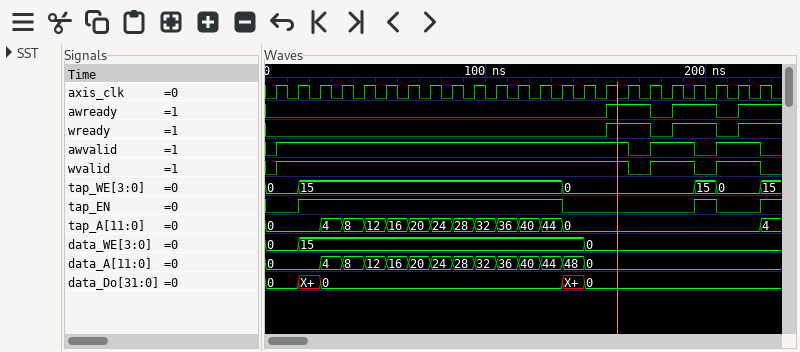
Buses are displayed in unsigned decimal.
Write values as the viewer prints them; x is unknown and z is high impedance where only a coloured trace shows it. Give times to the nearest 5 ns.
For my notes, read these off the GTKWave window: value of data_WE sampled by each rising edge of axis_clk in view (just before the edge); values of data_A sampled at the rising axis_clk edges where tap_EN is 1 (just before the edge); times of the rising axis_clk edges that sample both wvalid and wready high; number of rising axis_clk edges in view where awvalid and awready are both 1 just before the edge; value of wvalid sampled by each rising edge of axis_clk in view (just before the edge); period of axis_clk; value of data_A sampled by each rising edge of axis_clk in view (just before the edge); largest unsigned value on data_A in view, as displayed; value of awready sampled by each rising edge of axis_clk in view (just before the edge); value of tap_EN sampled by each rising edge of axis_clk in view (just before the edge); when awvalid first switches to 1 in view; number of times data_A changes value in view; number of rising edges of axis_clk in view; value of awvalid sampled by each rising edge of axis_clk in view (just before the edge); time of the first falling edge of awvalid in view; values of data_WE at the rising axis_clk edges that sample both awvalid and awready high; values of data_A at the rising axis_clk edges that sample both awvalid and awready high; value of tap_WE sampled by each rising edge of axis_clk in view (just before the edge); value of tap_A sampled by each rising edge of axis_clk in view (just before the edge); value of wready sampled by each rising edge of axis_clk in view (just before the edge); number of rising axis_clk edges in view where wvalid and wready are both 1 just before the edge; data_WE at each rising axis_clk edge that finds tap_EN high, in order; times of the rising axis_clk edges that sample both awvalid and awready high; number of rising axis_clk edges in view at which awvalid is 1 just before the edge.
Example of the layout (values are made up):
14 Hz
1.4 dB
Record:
0, 0, 15, 15, 15, 15, 15, 15, 15, 15, 15, 15, 15, 15, 15, 0, 0, 0, 0, 0, 0, 0, 0
0, 4, 8, 12, 16, 20, 24, 28, 32, 36, 40, 44, 0
165 ns, 195 ns, 225 ns
3
0 1 1 1 1 1 1 1 1 1 1 1 1 1 1 1 1 0 1 1 0 1 1
10 ns
0, 0, 0, 4, 8, 12, 16, 20, 24, 28, 32, 36, 40, 44, 48, 0, 0, 0, 0, 0, 0, 0, 0
48
0 0 0 0 0 0 0 0 0 0 0 0 0 0 0 0 1 1 0 1 1 0 1
0 0 1 1 1 1 1 1 1 1 1 1 1 1 0 0 0 0 0 0 1 0 0
5 ns
13
23
0 1 1 1 1 1 1 1 1 1 1 1 1 1 1 1 1 0 1 1 0 1 1
165 ns
0, 0, 0
0, 0, 0
0, 0, 15, 15, 15, 15, 15, 15, 15, 15, 15, 15, 15, 15, 0, 0, 0, 0, 0, 0, 15, 0, 0
0, 0, 0, 4, 8, 12, 16, 20, 24, 28, 32, 36, 40, 44, 0, 0, 0, 0, 0, 0, 0, 0, 0
0 0 0 0 0 0 0 0 0 0 0 0 0 0 0 0 1 1 0 1 1 0 1
3
15, 15, 15, 15, 15, 15, 15, 15, 15, 15, 15, 15, 0
165 ns, 195 ns, 225 ns
20
